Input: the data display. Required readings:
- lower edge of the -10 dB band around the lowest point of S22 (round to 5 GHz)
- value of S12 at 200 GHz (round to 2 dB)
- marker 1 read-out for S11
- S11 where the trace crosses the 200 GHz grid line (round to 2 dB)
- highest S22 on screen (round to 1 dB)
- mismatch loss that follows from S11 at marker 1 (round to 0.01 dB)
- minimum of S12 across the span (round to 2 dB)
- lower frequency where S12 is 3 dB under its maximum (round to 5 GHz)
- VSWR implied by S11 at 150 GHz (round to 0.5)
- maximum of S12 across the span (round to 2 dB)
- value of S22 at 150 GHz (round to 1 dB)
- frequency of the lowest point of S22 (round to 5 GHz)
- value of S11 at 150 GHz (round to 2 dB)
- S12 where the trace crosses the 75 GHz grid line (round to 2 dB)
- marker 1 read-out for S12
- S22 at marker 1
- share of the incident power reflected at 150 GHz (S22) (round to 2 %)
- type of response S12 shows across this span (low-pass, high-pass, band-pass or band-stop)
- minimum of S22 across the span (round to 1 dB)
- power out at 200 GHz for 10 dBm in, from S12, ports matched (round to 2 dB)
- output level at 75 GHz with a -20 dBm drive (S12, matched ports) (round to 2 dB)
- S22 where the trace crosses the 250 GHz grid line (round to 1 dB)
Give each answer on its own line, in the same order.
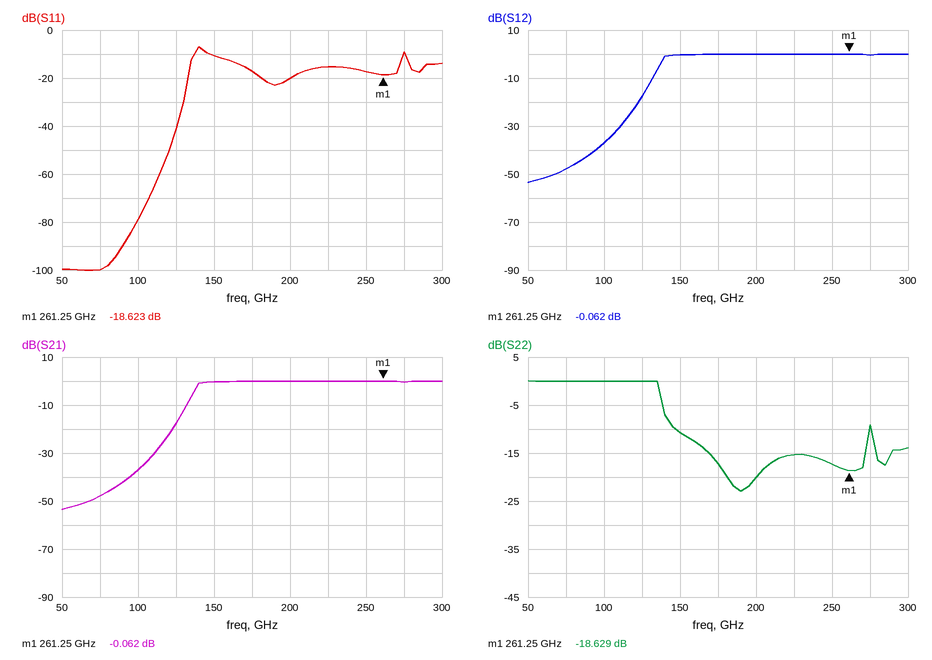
145 GHz
0 dB
-18.623 dB
-20 dB
0 dB
0.06 dB
-54 dB
140 GHz
2.0
0 dB
-11 dB
190 GHz
-10 dB
-48 dB
-0.062 dB
-18.629 dB
8 %
high-pass
-23 dB
10 dBm
-68 dBm
-17 dB
